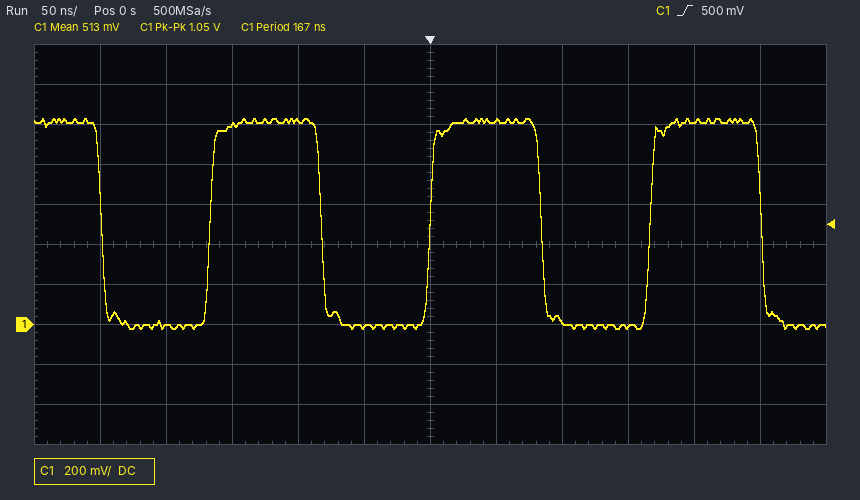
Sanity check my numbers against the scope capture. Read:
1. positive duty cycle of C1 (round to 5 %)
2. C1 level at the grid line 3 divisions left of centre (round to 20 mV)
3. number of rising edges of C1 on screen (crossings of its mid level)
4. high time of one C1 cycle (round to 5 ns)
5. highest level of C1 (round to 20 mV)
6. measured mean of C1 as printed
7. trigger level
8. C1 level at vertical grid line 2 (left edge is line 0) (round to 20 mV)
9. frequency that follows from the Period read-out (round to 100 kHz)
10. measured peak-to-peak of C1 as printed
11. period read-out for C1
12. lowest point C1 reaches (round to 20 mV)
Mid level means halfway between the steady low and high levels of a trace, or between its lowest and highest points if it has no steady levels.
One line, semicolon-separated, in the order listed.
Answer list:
50 %; 1.00 V; 3; 85 ns; 1.04 V; 513 mV; 500 mV; 0 mV; 6.0 MHz; 1.05 V; 167 ns; -20 mV
